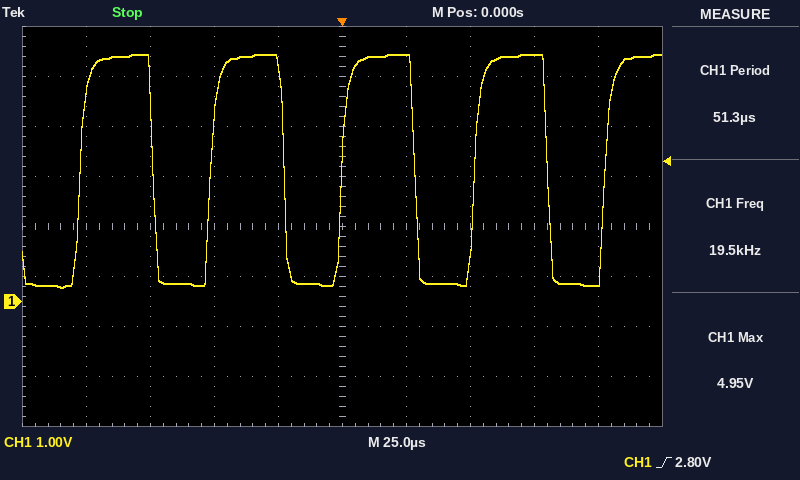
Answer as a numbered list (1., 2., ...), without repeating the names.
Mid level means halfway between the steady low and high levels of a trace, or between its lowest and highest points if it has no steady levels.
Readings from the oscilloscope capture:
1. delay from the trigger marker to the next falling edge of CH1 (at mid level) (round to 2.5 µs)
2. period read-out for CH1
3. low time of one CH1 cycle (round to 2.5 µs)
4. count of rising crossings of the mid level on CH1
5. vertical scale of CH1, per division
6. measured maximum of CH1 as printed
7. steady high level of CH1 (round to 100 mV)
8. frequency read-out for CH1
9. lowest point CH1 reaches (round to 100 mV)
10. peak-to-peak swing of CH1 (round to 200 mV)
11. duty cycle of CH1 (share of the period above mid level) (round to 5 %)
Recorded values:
1. 27.5 µs
2. 51.3 µs
3. 22.5 µs
4. 5
5. 1 V
6. 4.95 V
7. 4.9 V
8. 19.5 kHz
9. 300 mV
10. 4.6 V
11. 55 %
